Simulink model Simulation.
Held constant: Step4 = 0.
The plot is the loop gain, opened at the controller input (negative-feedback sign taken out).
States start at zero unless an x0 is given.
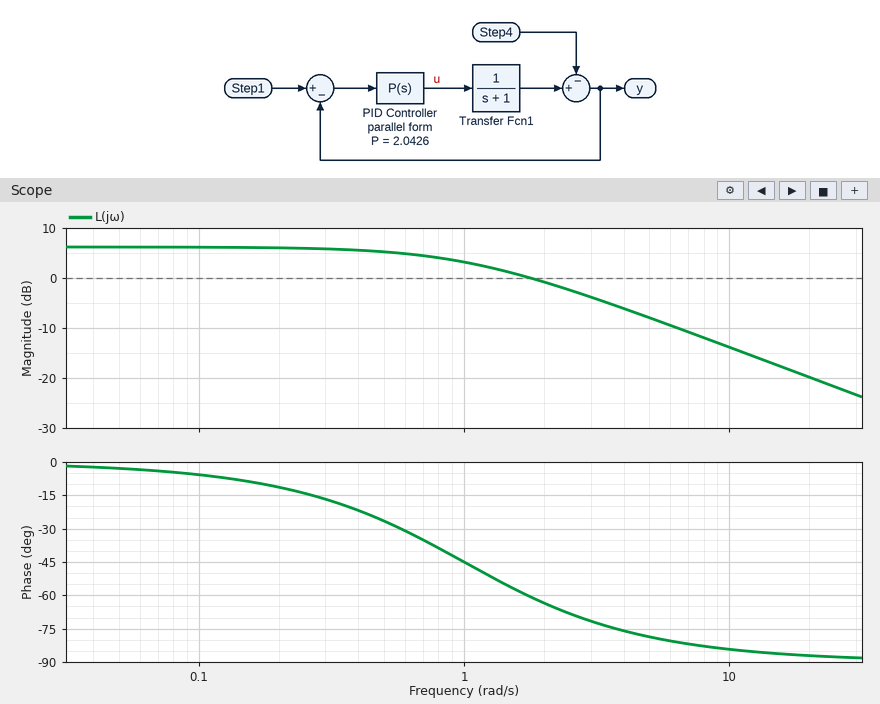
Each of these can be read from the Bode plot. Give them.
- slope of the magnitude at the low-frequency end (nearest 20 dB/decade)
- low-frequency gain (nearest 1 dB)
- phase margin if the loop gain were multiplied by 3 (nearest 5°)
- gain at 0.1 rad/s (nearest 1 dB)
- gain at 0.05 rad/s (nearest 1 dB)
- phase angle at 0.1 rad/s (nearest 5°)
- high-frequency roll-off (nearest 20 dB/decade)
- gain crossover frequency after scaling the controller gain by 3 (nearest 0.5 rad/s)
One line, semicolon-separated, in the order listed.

0 dB/decade; 6 dB; 100°; 6 dB; 6 dB; -5°; -20 dB/decade; 6.0 rad/s
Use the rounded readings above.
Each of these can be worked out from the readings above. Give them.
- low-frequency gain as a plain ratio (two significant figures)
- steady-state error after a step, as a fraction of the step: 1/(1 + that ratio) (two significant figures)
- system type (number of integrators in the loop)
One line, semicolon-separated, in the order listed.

2.0; 0.33; 0
